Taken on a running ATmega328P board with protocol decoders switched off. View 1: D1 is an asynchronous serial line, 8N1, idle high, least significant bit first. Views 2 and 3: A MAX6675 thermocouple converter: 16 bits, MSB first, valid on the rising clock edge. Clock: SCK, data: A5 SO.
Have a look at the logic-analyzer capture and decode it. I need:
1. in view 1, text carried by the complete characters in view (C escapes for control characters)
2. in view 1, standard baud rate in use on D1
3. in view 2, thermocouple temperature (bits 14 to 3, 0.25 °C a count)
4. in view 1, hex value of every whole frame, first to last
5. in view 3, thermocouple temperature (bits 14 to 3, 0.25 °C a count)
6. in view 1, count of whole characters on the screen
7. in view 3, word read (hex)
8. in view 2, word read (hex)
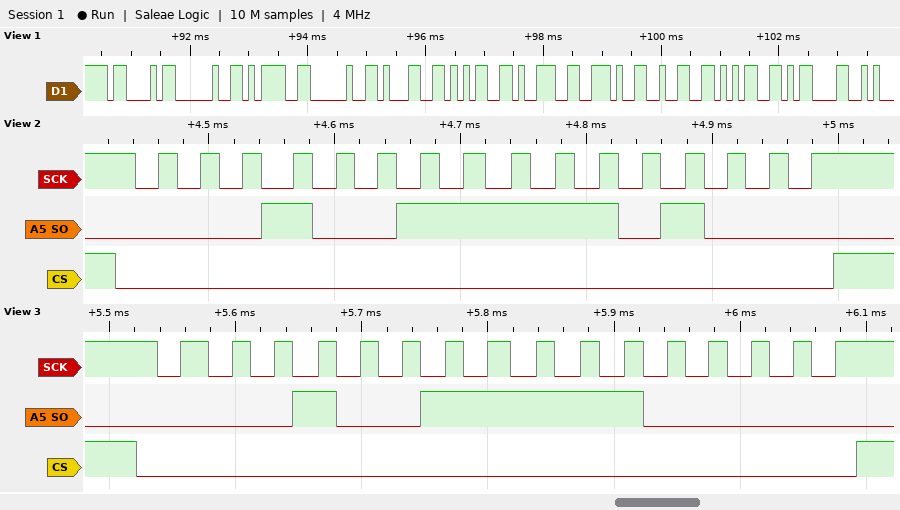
"C = 159.25\r"
9600 baud
159.25 °C
43 20 3D 20 31 35 39 2E 32 35 0D
159.00 °C
11
0x13E0
0x13E8
